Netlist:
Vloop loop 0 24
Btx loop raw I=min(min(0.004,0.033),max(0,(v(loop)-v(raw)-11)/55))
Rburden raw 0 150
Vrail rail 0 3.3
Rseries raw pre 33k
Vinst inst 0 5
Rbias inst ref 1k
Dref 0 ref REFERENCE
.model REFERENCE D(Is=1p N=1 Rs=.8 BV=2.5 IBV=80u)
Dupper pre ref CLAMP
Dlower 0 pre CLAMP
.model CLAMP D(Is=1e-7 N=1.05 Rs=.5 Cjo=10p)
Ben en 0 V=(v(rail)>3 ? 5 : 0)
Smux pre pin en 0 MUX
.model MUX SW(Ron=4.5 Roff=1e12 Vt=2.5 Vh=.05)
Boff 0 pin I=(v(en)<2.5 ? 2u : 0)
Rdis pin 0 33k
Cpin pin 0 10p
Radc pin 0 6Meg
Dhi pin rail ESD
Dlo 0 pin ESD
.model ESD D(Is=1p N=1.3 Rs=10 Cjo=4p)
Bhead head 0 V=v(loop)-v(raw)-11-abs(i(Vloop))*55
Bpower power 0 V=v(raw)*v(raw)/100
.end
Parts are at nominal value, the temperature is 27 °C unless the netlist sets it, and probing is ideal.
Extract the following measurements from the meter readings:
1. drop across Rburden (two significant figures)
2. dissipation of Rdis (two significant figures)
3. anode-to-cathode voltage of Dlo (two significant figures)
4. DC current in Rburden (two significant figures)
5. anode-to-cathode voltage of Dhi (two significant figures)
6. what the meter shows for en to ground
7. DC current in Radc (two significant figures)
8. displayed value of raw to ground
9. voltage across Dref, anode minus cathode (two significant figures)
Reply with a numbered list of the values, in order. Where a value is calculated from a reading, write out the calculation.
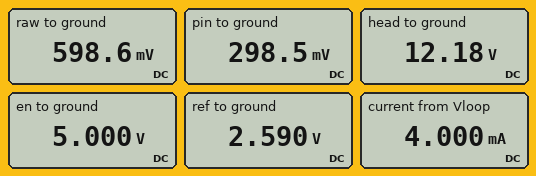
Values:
1. 598.6 mV = 600 mV
2. (298.5 mV)^2 / 33 kΩ = 2.7 µW
3. 0 V - 298.5 mV = -300 mV
4. (598.6 mV) / 150 Ω = 4.0 mA
5. 298.5 mV - 3.3 V = -3.0 V
6. 5.000 V
7. (298.5 mV) / 6 MΩ = 50 nA
8. 598.6 mV
9. 0 V - 2.59 V = -2.6 V
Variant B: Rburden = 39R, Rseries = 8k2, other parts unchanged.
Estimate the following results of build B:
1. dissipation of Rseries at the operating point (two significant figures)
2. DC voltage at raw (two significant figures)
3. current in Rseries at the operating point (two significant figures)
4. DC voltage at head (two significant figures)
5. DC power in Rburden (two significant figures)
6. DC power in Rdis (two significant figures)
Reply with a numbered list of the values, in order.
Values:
1. 120 nW
2. 160 mV
3. 3.8 µA
4. 13 V
5. 620 µW
6. 470 nW
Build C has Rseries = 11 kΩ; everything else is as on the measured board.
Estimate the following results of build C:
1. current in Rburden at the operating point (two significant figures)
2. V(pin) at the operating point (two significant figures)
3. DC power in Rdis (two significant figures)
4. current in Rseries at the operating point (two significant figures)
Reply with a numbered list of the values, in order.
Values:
1. 4.0 mA
2. 450 mV
3. 6.1 µW
4. 14 µA
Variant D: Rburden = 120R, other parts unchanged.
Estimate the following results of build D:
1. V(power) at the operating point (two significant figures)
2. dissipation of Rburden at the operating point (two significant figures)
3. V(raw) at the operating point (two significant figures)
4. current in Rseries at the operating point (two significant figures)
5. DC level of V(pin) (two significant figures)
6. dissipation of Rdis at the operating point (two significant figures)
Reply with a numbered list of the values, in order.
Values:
1. 2.3 mV
2. 1.9 mW
3. 480 mV
4. 7.3 µA
5. 240 mV
6. 1.7 µW
